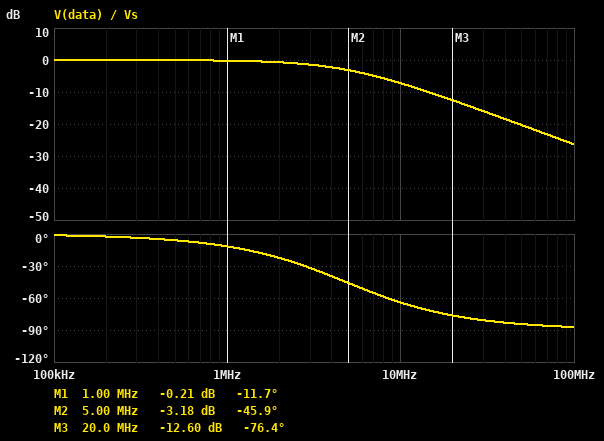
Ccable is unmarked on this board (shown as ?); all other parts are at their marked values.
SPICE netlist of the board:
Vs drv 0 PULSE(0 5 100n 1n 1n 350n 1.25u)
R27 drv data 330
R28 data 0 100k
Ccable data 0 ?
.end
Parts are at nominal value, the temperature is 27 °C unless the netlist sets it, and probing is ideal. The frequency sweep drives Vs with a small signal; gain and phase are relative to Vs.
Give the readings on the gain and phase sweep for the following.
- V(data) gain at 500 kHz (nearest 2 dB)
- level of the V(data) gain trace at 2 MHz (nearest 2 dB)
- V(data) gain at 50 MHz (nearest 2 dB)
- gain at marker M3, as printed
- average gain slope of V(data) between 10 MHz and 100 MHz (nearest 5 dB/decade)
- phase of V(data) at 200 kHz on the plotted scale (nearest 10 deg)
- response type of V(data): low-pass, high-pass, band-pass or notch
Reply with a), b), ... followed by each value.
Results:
a) 0 dB
b) 0 dB
c) -20 dB
d) -12.60 dB
e) -20 dB/decade
f) 0 deg
g) low-pass
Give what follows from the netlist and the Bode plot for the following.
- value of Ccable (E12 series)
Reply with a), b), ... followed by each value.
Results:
a) 100 pF
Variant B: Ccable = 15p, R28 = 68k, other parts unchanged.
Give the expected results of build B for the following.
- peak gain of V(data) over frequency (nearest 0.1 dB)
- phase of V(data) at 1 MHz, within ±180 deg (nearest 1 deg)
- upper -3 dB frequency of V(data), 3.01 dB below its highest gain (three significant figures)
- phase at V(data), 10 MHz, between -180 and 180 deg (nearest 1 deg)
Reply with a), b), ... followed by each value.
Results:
a) 0 dB
b) -2 deg
c) 32.3 MHz
d) -17 deg
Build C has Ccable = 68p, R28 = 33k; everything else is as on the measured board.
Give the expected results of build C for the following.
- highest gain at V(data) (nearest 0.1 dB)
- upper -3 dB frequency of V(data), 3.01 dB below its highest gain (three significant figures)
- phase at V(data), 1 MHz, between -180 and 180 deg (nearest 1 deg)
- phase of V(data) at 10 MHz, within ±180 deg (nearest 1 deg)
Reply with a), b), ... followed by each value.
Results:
a) -0.1 dB
b) 7.16 MHz
c) -8 deg
d) -54 deg
